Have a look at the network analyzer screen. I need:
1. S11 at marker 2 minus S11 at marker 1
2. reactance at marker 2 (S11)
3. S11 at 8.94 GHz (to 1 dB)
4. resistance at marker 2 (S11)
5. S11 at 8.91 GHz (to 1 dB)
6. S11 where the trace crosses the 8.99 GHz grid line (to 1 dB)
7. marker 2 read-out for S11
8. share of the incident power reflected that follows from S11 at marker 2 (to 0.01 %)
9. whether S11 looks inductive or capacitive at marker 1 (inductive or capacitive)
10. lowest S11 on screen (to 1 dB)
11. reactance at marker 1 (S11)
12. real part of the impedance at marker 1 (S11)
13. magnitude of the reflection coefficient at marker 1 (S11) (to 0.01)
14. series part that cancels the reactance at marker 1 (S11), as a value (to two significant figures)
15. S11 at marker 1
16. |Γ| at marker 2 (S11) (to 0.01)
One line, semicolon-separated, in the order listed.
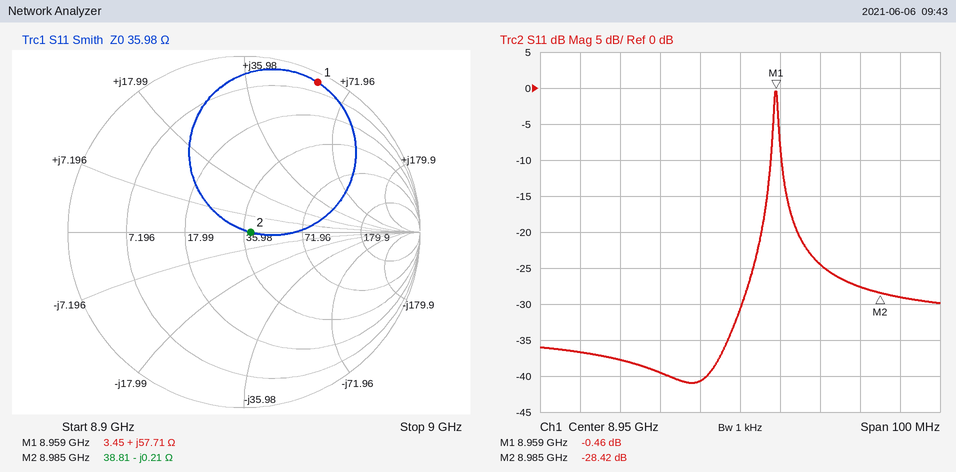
-27.96 dB; -0.21 Ω; -41 dB; 38.81 Ω; -37 dB; -29 dB; -28.42 dB; 0.14 %; inductive; -41 dB; +57.71 Ω; 3.45 Ω; 0.95; 310 fF; -0.46 dB; 0.04
